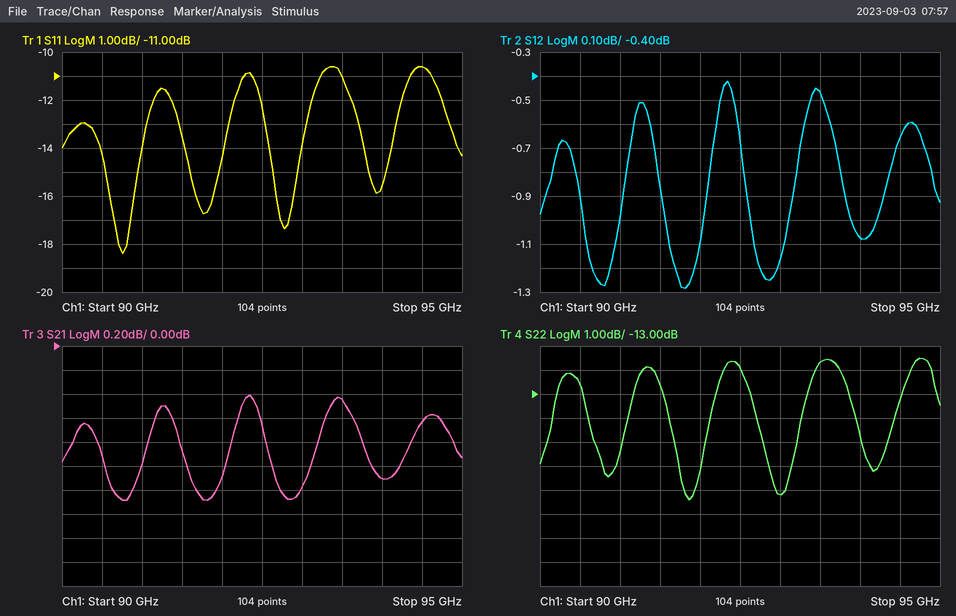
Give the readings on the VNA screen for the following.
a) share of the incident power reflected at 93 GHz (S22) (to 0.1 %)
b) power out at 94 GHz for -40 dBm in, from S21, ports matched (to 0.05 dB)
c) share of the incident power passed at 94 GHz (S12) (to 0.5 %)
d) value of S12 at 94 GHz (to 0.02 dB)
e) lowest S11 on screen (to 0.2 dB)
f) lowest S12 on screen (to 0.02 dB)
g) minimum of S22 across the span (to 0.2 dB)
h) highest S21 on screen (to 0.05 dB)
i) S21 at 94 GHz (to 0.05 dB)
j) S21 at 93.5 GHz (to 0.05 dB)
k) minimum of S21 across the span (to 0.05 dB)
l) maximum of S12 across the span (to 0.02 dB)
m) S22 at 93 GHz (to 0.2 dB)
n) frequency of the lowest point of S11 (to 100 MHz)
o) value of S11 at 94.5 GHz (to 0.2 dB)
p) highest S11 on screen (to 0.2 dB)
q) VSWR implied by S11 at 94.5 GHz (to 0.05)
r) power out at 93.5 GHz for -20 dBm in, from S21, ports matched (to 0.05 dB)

1.9 %
-41.10 dBm
78.0 %
-1.08 dB
-18.4 dB
-1.28 dB
-17.4 dB
-0.40 dB
-1.10 dB
-0.45 dB
-1.30 dB
-0.42 dB
-17.2 dB
90.8 GHz
-10.6 dB
-10.6 dB
1.85
-20.45 dBm
